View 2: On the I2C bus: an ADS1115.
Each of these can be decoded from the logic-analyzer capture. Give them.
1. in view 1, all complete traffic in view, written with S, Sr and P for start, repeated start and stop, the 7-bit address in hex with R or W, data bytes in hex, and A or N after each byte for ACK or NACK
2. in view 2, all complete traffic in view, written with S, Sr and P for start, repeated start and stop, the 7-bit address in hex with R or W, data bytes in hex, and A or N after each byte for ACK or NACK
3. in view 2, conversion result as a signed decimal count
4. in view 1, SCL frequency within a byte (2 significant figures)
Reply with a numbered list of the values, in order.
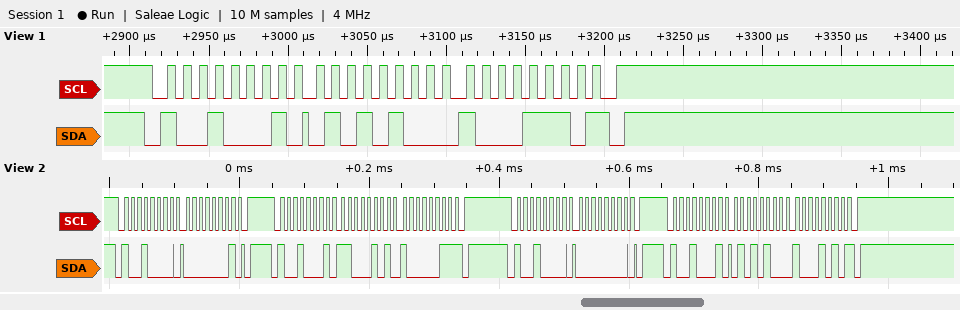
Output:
1. S 48R A 54 A 8E N P
2. S 48W A 01 A P S 48R A C5 A 83 N P S 48W A 00 A P S 48R A 54 A 8A N P
3. 21642
4. 100 kHz
